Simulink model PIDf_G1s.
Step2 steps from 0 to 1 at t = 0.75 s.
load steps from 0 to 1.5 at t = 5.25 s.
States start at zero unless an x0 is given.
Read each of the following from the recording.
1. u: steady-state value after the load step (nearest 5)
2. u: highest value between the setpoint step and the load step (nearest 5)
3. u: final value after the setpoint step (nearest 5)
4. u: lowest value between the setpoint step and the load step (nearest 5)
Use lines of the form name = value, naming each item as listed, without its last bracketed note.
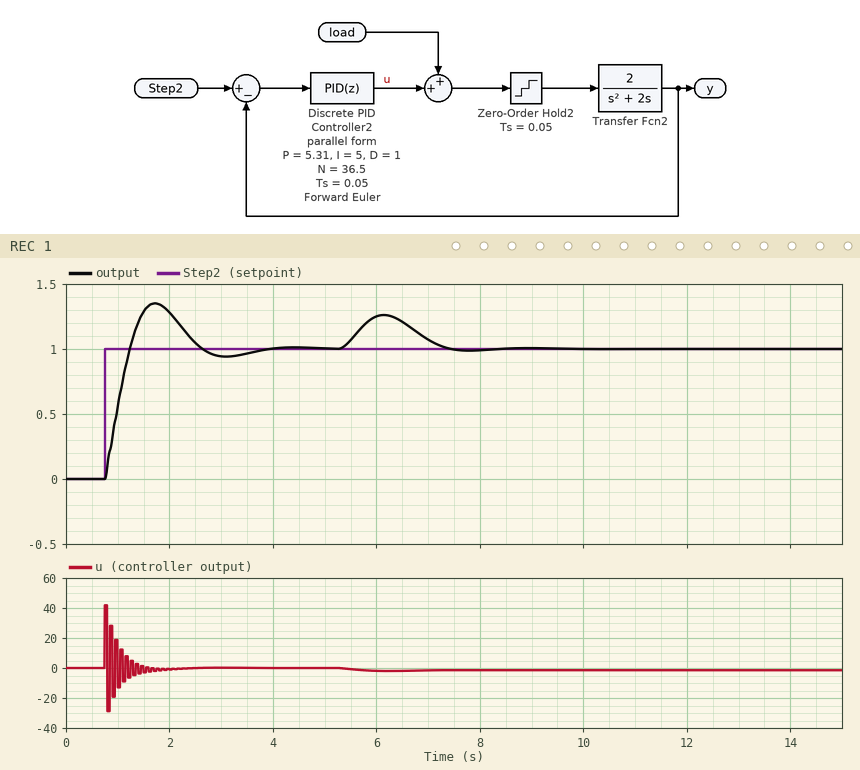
u: steady-state value after the load step = 0
u: highest value between the setpoint step and the load step = 40
u: final value after the setpoint step = 0
u: lowest value between the setpoint step and the load step = -30
